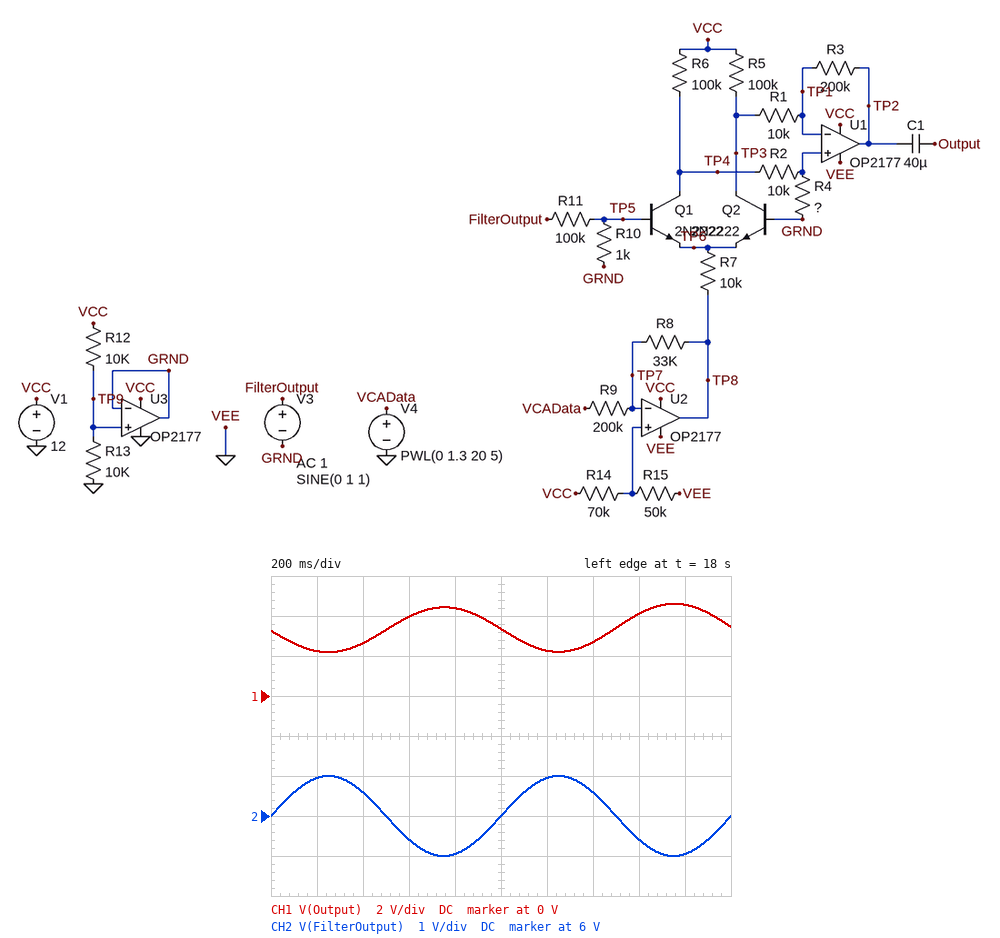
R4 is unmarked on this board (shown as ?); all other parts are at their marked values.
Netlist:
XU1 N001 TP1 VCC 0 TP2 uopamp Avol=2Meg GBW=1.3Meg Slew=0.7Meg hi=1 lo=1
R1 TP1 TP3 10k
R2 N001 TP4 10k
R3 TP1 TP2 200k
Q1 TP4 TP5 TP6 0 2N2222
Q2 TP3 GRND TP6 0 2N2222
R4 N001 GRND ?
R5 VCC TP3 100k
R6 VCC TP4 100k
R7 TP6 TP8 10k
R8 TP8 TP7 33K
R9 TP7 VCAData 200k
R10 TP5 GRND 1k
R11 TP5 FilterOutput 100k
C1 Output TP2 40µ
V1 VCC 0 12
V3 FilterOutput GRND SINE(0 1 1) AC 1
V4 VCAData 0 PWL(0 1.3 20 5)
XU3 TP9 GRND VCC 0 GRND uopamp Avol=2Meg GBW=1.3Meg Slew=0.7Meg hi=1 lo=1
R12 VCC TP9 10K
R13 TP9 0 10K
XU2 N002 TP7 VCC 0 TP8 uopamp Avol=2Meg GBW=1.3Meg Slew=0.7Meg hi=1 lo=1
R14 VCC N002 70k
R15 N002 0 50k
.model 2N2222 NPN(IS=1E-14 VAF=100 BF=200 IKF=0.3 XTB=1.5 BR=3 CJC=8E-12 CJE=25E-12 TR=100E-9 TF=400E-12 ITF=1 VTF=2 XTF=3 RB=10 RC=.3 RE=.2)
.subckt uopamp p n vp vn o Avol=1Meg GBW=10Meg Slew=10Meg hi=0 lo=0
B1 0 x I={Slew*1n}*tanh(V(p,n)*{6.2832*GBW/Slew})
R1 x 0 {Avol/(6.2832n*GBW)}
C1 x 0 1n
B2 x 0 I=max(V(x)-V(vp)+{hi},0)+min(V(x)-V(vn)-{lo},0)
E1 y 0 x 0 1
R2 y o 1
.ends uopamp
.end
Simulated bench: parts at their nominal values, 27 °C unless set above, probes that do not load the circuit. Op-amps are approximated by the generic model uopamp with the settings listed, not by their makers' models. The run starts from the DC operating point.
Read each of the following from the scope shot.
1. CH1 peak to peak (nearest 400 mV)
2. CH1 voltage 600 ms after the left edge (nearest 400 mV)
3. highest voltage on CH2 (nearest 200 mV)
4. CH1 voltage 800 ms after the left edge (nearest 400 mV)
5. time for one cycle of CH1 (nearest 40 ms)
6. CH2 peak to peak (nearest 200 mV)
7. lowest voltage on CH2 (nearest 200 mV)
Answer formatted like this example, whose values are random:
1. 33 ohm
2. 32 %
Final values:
1. 2.4 V
2. 4.0 V
3. 7.0 V
4. 4.4 V
5. 1.00 s
6. 2.0 V
7. 5.0 V
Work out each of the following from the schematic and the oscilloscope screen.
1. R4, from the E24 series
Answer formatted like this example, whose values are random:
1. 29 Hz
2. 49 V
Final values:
1. 75 kΩ
